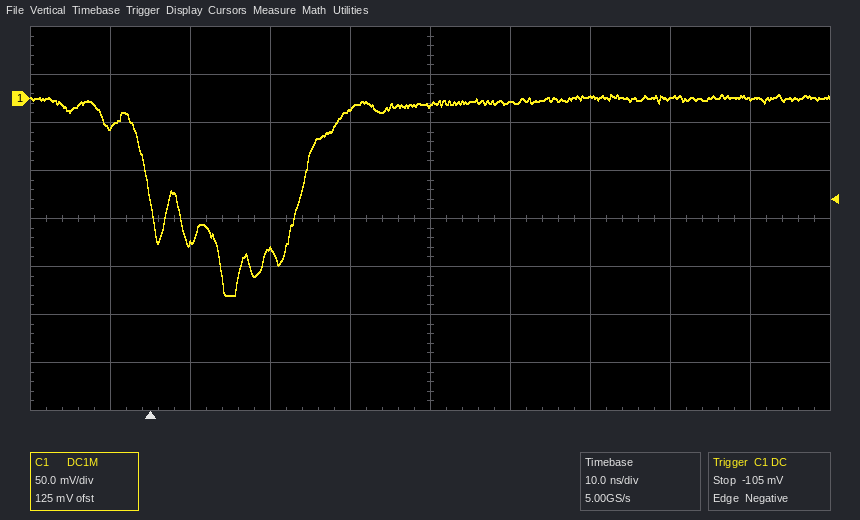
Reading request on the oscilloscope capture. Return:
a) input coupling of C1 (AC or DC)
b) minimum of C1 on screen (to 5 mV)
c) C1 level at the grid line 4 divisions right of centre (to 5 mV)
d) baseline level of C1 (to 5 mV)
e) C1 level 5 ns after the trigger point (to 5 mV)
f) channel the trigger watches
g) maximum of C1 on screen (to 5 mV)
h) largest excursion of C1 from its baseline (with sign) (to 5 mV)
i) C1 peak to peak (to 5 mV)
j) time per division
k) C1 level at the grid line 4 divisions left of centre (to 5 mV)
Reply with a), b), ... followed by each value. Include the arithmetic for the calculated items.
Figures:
a) DC
b) -205 mV
c) 0 mV
d) 0 mV
e) -150 mV
f) C1
g) 5 mV
h) -205 mV − (0 mV) = -205 mV
i) 5 mV − (-205 mV) = 210 mV
j) 10 ns
k) -30 mV
